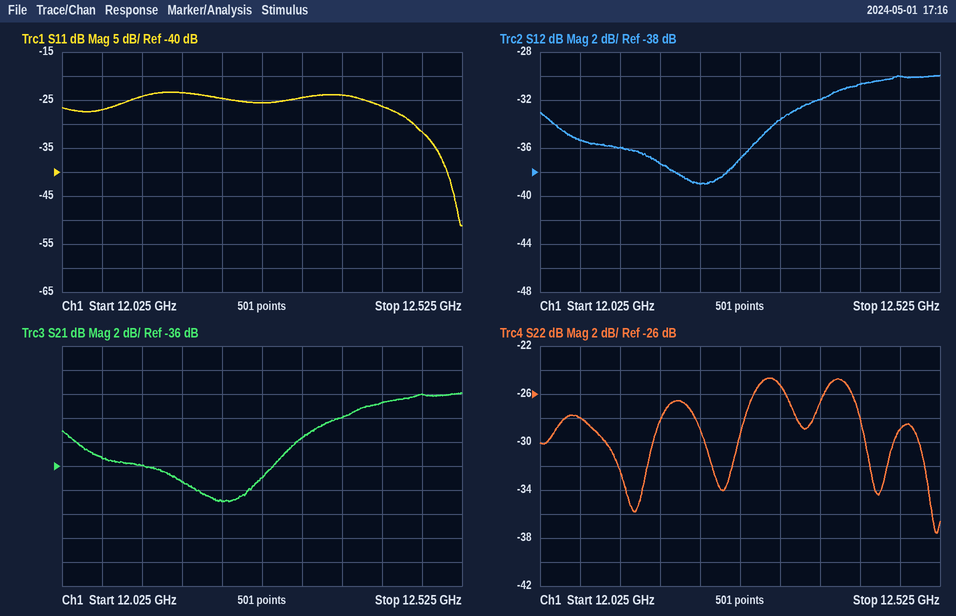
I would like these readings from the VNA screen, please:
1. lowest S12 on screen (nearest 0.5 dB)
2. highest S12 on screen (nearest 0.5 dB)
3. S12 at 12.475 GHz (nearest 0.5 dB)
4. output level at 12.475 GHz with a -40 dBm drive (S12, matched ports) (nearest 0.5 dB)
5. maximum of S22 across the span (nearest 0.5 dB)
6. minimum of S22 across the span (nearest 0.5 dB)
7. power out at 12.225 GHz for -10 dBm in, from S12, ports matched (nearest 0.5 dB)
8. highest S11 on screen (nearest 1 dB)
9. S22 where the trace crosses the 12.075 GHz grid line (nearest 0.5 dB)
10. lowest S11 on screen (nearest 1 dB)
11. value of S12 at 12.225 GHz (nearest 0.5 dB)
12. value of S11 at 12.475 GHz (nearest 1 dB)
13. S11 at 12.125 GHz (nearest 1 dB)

-39.0 dB
-30.0 dB
-30.0 dB
-70.0 dBm
-24.5 dB
-37.5 dB
-49.0 dBm
-23 dB
-28.0 dB
-51 dB
-39.0 dB
-32 dB
-24 dB
